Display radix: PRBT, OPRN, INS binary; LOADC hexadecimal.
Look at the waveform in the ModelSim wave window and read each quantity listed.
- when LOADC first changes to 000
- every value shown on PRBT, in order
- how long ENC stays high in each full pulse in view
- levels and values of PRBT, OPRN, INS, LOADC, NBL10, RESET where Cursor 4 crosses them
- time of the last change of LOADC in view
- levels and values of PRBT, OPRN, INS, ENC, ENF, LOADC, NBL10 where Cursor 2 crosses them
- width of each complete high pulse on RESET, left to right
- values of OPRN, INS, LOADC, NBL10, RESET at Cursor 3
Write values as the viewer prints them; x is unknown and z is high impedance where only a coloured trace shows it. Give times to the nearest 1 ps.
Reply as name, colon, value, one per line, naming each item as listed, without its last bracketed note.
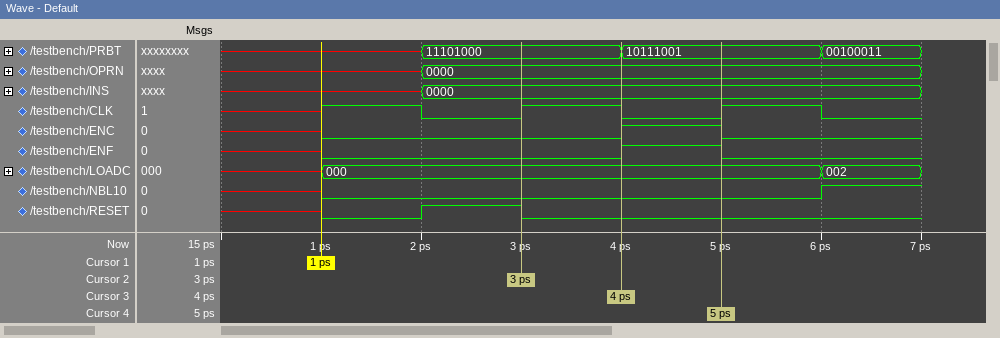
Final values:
when LOADC first changes to 000: 1 ps
every value shown on PRBT, in order: x, 11101000, 10111001, 00100011
how long ENC stays high in each full pulse in view: 1 ps
levels and values of PRBT, OPRN, INS, LOADC, NBL10, RESET where Cursor 4 crosses them: PRBT=10111001, OPRN=0000, INS=0000, LOADC=000, NBL10=0, RESET=0
time of the last change of LOADC in view: 6 ps
levels and values of PRBT, OPRN, INS, ENC, ENF, LOADC, NBL10 where Cursor 2 crosses them: PRBT=11101000, OPRN=0000, INS=0000, ENC=0, ENF=0, LOADC=000, NBL10=0
width of each complete high pulse on RESET, left to right: 1 ps
values of OPRN, INS, LOADC, NBL10, RESET at Cursor 3: OPRN=0000, INS=0000, LOADC=000, NBL10=0, RESET=0
